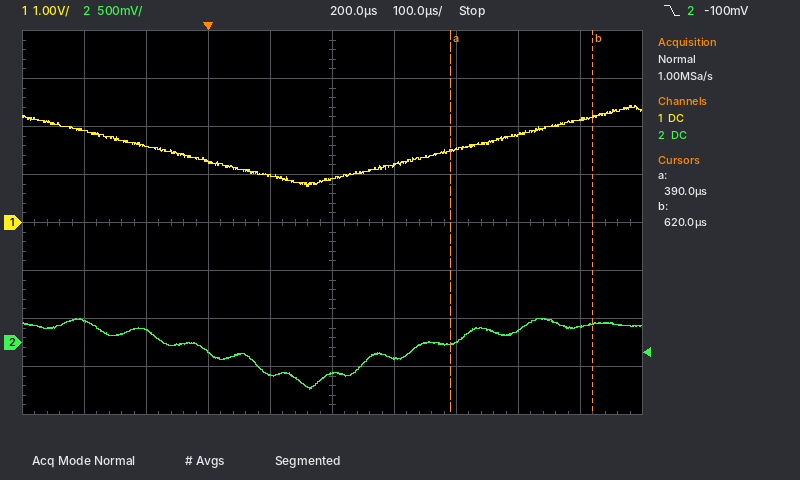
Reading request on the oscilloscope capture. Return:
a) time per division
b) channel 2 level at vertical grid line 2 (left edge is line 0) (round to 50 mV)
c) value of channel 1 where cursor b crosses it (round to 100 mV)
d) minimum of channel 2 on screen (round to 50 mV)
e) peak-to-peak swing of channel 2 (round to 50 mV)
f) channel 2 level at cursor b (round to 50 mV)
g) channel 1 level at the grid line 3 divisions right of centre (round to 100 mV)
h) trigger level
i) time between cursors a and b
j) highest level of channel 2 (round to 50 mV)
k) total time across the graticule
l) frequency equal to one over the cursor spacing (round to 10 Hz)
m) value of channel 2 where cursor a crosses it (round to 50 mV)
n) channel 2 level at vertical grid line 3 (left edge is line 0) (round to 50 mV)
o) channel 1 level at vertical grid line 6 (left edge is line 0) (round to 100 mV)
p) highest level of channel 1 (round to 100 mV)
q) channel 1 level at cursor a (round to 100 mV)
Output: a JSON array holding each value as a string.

["100 µs", "150 mV", "2.2 V", "-500 mV", "750 mV", "200 mV", "1.8 V", "-100 mV", "230 µs", "250 mV", "1 ms", "4.35 kHz", "0 mV", "-100 mV", "1.2 V", "2.4 V", "1.5 V"]
